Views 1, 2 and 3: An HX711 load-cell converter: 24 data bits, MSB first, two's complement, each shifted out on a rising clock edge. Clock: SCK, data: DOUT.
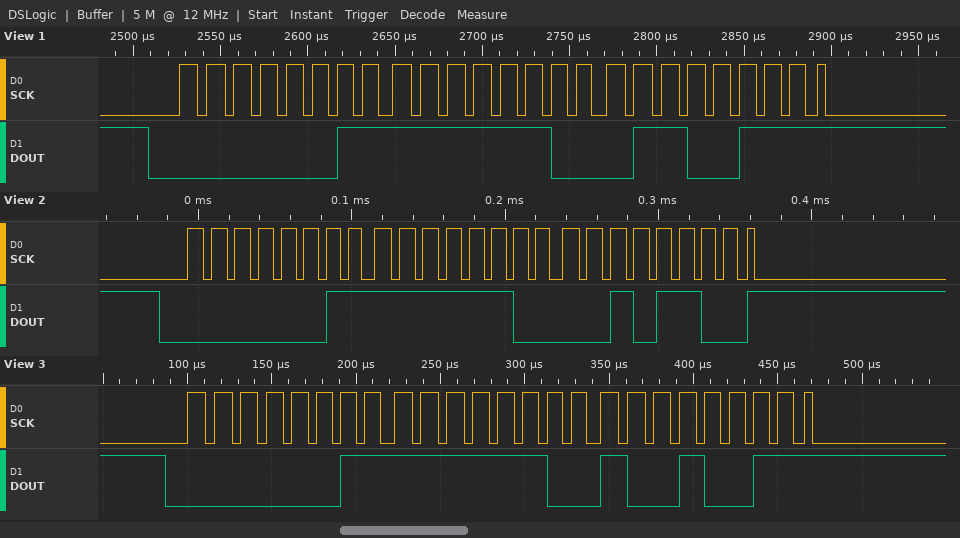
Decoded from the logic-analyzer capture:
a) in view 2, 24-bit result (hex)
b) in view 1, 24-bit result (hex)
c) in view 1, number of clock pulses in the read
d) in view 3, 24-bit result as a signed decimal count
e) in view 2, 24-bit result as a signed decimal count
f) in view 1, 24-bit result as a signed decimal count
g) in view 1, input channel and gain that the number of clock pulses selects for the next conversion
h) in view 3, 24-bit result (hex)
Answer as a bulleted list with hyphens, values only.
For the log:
- 0x03FC2C
- 0x03FC67
- 25
- 261267
- 261164
- 261223
- channel A, gain 128
- 0x03FC93
